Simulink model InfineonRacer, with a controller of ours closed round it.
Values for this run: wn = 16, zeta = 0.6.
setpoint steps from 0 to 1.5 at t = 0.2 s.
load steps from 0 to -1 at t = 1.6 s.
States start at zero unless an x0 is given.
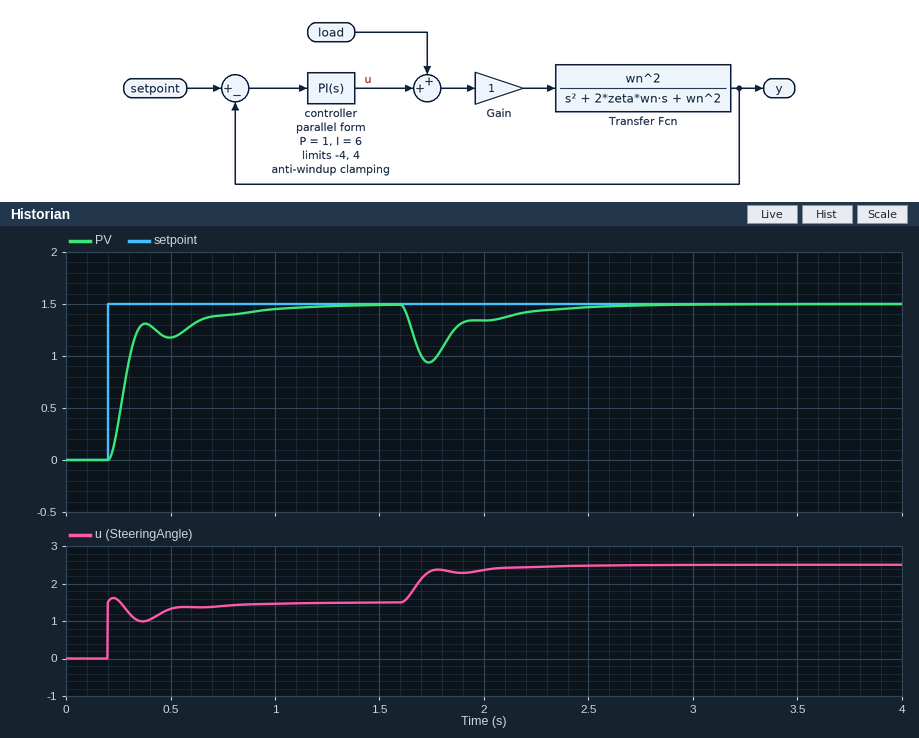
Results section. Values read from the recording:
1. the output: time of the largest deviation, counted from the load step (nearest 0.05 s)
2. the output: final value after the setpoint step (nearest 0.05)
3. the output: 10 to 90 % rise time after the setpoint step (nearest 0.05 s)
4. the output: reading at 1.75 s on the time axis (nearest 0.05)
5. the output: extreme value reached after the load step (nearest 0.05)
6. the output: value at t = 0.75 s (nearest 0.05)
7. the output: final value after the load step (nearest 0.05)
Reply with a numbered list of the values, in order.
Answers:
1. 0.15 s
2. 1.50
3. 0.40 s
4. 0.95
5. 0.95
6. 1.40
7. 1.50
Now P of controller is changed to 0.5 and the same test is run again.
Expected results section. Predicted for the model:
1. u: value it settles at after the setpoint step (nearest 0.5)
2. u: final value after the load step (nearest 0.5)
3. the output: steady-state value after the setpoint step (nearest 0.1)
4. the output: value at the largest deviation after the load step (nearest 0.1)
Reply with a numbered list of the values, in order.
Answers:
1. 1.5
2. 2.5
3. 1.5
4. 0.8
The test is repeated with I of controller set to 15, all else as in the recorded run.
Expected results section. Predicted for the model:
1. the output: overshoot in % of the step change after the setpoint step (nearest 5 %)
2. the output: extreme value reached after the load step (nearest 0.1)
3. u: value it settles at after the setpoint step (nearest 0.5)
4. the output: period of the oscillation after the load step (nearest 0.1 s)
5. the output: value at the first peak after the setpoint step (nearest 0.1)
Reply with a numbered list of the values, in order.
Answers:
1. 20 %
2. 1.0
3. 1.5
4. 0.3 s
5. 1.8
